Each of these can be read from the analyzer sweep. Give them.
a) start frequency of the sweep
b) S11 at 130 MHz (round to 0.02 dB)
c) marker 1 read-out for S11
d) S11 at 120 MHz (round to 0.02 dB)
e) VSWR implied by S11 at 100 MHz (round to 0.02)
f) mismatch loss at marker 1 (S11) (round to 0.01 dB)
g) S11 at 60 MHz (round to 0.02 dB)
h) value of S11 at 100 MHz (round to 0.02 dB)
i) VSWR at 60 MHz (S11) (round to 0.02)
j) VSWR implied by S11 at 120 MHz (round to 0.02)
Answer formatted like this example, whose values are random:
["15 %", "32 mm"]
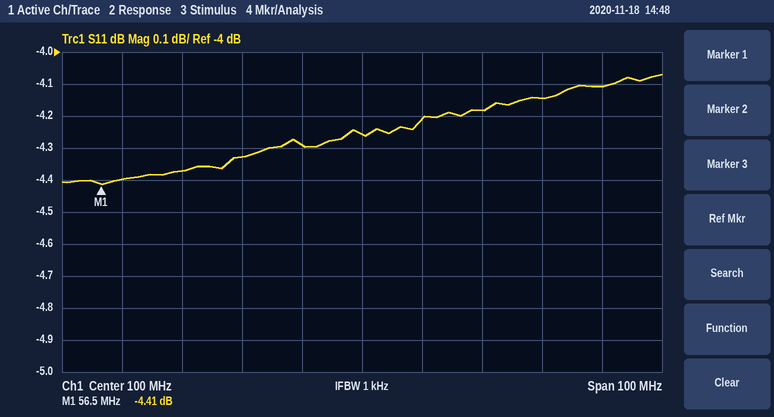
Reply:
["50 MHz", "-4.14 dB", "-4.41 dB", "-4.18 dB", "4.16", "1.95 dB", "-4.40 dB", "-4.26 dB", "4.04", "4.24"]
